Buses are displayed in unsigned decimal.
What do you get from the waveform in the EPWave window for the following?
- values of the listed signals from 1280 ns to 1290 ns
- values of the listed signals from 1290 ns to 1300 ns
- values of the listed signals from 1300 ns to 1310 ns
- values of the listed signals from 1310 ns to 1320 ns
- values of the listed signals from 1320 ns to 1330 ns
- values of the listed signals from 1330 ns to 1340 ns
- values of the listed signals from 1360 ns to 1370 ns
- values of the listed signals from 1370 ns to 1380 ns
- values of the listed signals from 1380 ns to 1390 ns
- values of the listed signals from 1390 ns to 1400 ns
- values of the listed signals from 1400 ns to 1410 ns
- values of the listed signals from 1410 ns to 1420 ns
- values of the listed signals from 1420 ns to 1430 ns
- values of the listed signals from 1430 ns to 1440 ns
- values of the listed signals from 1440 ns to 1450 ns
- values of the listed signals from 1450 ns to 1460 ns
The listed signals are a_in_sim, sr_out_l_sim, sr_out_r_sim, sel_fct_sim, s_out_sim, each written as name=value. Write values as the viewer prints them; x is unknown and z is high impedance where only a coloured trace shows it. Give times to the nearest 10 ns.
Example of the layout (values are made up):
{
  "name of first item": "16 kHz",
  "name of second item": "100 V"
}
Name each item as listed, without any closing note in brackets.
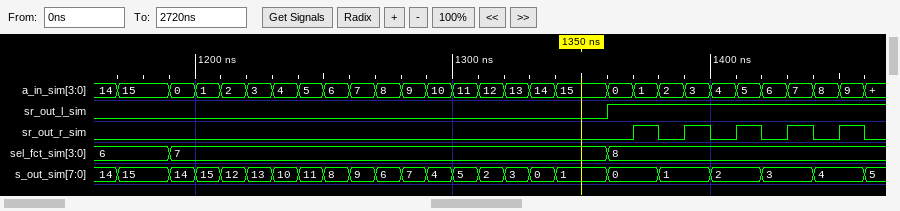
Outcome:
{
  "values of the listed signals from 1280 ns to 1290 ns": "a_in_sim=9, sr_out_l_sim=0, sr_out_r_sim=0, sel_fct_sim=7, s_out_sim=7",
  "values of the listed signals from 1290 ns to 1300 ns": "a_in_sim=10, sr_out_l_sim=0, sr_out_r_sim=0, sel_fct_sim=7, s_out_sim=4",
  "values of the listed signals from 1300 ns to 1310 ns": "a_in_sim=11, sr_out_l_sim=0, sr_out_r_sim=0, sel_fct_sim=7, s_out_sim=5",
  "values of the listed signals from 1310 ns to 1320 ns": "a_in_sim=12, sr_out_l_sim=0, sr_out_r_sim=0, sel_fct_sim=7, s_out_sim=2",
  "values of the listed signals from 1320 ns to 1330 ns": "a_in_sim=13, sr_out_l_sim=0, sr_out_r_sim=0, sel_fct_sim=7, s_out_sim=3",
  "values of the listed signals from 1330 ns to 1340 ns": "a_in_sim=14, sr_out_l_sim=0, sr_out_r_sim=0, sel_fct_sim=7, s_out_sim=0",
  "values of the listed signals from 1360 ns to 1370 ns": "a_in_sim=0, sr_out_l_sim=1, sr_out_r_sim=0, sel_fct_sim=8, s_out_sim=0",
  "values of the listed signals from 1370 ns to 1380 ns": "a_in_sim=1, sr_out_l_sim=1, sr_out_r_sim=1, sel_fct_sim=8, s_out_sim=0",
  "values of the listed signals from 1380 ns to 1390 ns": "a_in_sim=2, sr_out_l_sim=1, sr_out_r_sim=0, sel_fct_sim=8, s_out_sim=1",
  "values of the listed signals from 1390 ns to 1400 ns": "a_in_sim=3, sr_out_l_sim=1, sr_out_r_sim=1, sel_fct_sim=8, s_out_sim=1",
  "values of the listed signals from 1400 ns to 1410 ns": "a_in_sim=4, sr_out_l_sim=1, sr_out_r_sim=0, sel_fct_sim=8, s_out_sim=2",
  "values of the listed signals from 1410 ns to 1420 ns": "a_in_sim=5, sr_out_l_sim=1, sr_out_r_sim=1, sel_fct_sim=8, s_out_sim=2",
  "values of the listed signals from 1420 ns to 1430 ns": "a_in_sim=6, sr_out_l_sim=1, sr_out_r_sim=0, sel_fct_sim=8, s_out_sim=3",
  "values of the listed signals from 1430 ns to 1440 ns": "a_in_sim=7, sr_out_l_sim=1, sr_out_r_sim=1, sel_fct_sim=8, s_out_sim=3",
  "values of the listed signals from 1440 ns to 1450 ns": "a_in_sim=8, sr_out_l_sim=1, sr_out_r_sim=0, sel_fct_sim=8, s_out_sim=4",
  "values of the listed signals from 1450 ns to 1460 ns": "a_in_sim=9, sr_out_l_sim=1, sr_out_r_sim=1, sel_fct_sim=8, s_out_sim=4"
}
